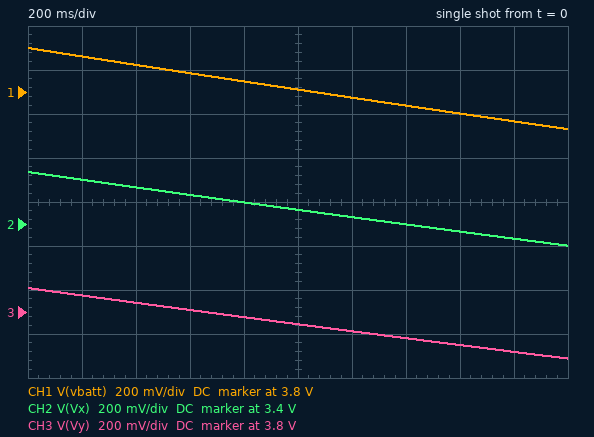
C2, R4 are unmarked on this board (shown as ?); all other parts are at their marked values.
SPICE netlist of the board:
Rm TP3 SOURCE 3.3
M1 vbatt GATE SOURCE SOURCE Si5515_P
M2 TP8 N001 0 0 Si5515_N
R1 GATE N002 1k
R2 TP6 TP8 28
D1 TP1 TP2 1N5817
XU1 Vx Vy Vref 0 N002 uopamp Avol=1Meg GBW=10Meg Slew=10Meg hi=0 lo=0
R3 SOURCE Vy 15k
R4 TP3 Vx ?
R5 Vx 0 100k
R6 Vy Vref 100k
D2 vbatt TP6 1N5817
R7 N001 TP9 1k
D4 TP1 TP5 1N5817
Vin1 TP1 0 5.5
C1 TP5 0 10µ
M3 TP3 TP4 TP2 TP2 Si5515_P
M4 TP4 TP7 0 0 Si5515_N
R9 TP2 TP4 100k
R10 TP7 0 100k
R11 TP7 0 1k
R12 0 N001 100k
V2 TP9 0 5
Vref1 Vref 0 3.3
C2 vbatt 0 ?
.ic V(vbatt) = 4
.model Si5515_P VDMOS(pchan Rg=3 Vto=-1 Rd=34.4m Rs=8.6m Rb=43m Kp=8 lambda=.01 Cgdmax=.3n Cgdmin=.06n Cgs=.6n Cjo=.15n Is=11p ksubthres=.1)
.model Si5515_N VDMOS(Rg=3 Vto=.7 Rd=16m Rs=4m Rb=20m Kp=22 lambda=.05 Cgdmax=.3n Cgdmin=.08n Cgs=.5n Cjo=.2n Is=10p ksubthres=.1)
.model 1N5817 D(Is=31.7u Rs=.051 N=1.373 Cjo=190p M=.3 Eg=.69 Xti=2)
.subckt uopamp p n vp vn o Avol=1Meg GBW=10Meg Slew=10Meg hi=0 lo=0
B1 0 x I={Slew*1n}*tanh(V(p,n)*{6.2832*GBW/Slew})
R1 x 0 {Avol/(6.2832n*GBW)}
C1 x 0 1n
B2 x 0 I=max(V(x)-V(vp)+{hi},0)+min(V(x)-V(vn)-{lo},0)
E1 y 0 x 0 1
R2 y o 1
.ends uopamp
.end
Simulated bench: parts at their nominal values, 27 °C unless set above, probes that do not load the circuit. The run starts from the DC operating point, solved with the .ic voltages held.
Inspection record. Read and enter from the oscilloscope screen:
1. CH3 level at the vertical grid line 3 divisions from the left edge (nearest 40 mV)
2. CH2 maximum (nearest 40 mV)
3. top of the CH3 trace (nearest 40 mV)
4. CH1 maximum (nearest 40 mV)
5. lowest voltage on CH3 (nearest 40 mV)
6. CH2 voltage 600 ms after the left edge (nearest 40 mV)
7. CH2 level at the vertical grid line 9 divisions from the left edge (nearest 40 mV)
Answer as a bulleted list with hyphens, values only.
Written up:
- 3.80 V
- 3.64 V
- 3.92 V
- 4.00 V
- 3.60 V
- 3.52 V
- 3.32 V
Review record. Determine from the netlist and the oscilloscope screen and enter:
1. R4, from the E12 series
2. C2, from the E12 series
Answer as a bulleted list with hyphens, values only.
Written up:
- 10 kΩ
- 680 mF
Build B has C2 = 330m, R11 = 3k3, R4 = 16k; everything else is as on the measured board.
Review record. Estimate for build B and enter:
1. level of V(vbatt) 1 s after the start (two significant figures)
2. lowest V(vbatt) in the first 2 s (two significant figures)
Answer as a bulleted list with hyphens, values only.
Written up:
- 3.6 V
- 3.3 V
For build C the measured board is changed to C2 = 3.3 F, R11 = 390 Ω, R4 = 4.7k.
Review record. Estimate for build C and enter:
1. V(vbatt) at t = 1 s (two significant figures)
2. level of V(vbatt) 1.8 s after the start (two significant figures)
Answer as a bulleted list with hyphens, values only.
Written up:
- 4.0 V
- 3.9 V
